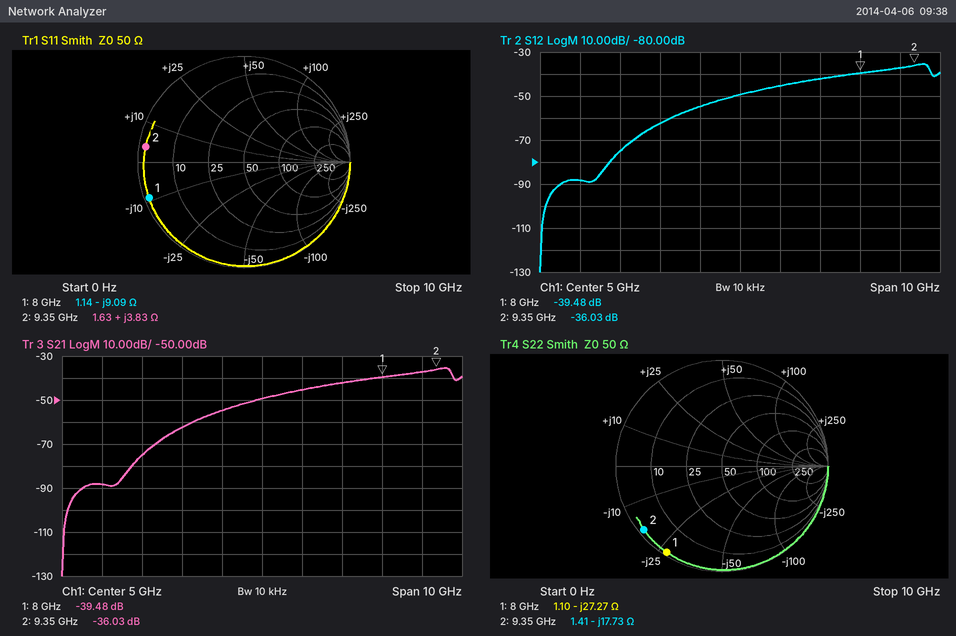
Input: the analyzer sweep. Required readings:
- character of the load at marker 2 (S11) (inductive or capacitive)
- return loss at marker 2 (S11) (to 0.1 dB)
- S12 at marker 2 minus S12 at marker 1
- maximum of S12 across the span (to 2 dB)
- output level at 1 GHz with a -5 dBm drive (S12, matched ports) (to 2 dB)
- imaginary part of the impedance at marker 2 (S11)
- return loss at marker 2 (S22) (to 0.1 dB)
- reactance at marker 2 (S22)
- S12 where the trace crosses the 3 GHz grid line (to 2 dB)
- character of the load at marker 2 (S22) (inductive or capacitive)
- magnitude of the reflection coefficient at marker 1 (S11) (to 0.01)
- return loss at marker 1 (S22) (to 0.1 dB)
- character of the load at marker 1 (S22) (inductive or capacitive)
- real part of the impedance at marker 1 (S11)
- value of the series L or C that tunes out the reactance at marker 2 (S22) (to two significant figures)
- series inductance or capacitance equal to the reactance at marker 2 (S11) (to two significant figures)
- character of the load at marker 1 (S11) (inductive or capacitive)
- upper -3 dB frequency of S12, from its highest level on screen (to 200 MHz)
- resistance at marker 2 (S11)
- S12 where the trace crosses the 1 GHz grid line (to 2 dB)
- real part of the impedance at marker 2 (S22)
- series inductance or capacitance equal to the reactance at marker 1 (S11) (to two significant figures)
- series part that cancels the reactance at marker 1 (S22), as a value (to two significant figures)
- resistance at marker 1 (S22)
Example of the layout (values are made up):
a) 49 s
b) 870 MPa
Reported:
a) inductive
b) 0.6 dB
c) 3.45 dB
d) -36 dB
e) -94 dBm
f) +3.83 Ω
g) 0.4 dB
h) -17.73 Ω
i) -62 dB
j) capacitive
k) 0.96
l) 0.3 dB
m) capacitive
n) 1.14 Ω
o) 300 pH
p) 65 pH
q) capacitive
r) 9.8 GHz
s) 1.63 Ω
t) -88 dB
u) 1.41 Ω
v) 2.2 pF
w) 540 pH
x) 1.10 Ω
